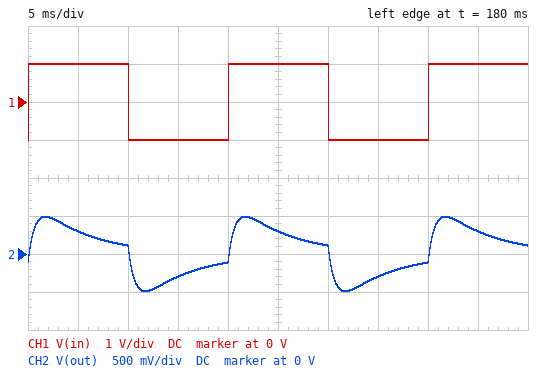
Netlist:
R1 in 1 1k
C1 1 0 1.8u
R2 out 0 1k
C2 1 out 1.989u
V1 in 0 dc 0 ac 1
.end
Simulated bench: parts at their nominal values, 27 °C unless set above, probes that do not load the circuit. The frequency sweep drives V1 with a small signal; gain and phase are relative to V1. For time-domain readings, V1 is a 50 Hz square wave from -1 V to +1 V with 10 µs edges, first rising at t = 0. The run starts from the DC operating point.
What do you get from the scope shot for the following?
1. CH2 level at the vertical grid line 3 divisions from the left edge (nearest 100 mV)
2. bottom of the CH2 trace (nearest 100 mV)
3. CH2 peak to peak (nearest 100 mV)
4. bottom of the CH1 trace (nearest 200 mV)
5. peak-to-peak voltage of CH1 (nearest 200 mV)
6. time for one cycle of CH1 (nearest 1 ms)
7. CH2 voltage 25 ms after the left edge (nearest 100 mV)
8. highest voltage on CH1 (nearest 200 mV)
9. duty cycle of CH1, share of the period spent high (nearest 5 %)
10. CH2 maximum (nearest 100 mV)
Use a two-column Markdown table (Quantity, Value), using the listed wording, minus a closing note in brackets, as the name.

| Quantity | Value |
|---|---|
| CH2 level at the vertical grid line 3 divisions from the left edge | -300 mV |
| bottom of the CH2 trace | -500 mV |
| CH2 peak to peak | 1.0 V |
| bottom of the CH1 trace | -1.0 V |
| peak-to-peak voltage of CH1 | 2.0 V |
| time for one cycle of CH1 | 20 ms |
| CH2 voltage 25 ms after the left edge | 300 mV |
| highest voltage on CH1 | 1.0 V |
| duty cycle of CH1, share of the period spent high | 50 % |
| CH2 maximum | 500 mV |
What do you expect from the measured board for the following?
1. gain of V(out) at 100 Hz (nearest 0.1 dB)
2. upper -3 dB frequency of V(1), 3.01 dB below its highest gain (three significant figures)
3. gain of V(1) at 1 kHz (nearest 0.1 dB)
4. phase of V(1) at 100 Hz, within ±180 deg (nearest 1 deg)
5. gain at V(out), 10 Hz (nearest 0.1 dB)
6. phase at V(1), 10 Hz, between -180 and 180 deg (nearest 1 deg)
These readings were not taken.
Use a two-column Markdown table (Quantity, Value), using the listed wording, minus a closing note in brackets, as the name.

| Quantity | Value |
|---|---|
| gain of V(out) at 100 Hz | -9.3 dB |
| upper -3 dB frequency of V(1), 3.01 dB below its highest gain | 36.5 Hz |
| gain of V(1) at 1 kHz | -21.3 dB |
| phase of V(1) at 100 Hz, within ±180 deg | -45 deg |
| gain at V(out), 10 Hz | -18.5 dB |
| phase at V(1), 10 Hz, between -180 and 180 deg | -13 deg |
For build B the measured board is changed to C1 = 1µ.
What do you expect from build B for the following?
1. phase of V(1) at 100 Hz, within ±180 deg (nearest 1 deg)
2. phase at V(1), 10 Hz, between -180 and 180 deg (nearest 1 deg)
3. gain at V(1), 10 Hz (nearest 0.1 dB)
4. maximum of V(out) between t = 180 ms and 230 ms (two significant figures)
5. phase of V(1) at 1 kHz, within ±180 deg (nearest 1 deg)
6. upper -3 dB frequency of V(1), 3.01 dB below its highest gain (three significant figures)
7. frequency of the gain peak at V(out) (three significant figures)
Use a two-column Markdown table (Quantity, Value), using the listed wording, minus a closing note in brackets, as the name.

| Quantity | Value |
|---|---|
| phase of V(1) at 100 Hz, within ±180 deg | -35 deg |
| phase at V(1), 10 Hz, between -180 and 180 deg | -10 deg |
| gain at V(1), 10 Hz | -0.3 dB |
| maximum of V(out) between t = 180 ms and 230 ms | 610 mV |
| phase of V(1) at 1 kHz, within ±180 deg | -73 deg |
| upper -3 dB frequency of V(1), 3.01 dB below its highest gain | 43.8 Hz |
| frequency of the gain peak at V(out) | 113 Hz |
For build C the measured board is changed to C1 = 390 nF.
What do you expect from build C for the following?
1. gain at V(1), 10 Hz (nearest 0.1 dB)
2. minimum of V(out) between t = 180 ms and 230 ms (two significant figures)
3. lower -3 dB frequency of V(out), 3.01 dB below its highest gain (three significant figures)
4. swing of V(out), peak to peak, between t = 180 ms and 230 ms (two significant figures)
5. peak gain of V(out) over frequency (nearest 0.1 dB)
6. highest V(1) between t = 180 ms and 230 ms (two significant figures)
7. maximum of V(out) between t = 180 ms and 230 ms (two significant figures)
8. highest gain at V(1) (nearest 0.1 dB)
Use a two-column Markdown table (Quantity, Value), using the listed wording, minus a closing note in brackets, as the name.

| Quantity | Value |
|---|---|
| gain at V(1), 10 Hz | -0.2 dB |
| minimum of V(out) between t = 180 ms and 230 ms | -750 mV |
| lower -3 dB frequency of V(out), 3.01 dB below its highest gain | 35.1 Hz |
| swing of V(out), peak to peak, between t = 180 ms and 230 ms | 1.5 V |
| peak gain of V(out) over frequency | -6.8 dB |
| highest V(1) between t = 180 ms and 230 ms | 910 mV |
| maximum of V(out) between t = 180 ms and 230 ms | 750 mV |
| highest gain at V(1) | 0 dB |
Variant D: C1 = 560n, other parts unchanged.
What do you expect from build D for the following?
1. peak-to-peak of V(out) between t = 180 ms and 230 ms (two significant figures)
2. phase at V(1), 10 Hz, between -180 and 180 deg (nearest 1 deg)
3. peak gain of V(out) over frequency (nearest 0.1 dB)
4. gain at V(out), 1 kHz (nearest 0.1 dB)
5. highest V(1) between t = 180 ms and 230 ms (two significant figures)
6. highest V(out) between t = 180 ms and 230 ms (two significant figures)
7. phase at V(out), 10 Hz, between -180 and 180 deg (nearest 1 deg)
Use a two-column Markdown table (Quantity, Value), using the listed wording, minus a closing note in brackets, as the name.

| Quantity | Value |
|---|---|
| peak-to-peak of V(out) between t = 180 ms and 230 ms | 1.4 V |
| phase at V(1), 10 Hz, between -180 and 180 deg | -9 deg |
| peak gain of V(out) over frequency | -7.2 dB |
| gain at V(out), 1 kHz | -12.3 dB |
| highest V(1) between t = 180 ms and 230 ms | 900 mV |
| highest V(out) between t = 180 ms and 230 ms | 700 mV |
| phase at V(out), 10 Hz, between -180 and 180 deg | 74 deg |
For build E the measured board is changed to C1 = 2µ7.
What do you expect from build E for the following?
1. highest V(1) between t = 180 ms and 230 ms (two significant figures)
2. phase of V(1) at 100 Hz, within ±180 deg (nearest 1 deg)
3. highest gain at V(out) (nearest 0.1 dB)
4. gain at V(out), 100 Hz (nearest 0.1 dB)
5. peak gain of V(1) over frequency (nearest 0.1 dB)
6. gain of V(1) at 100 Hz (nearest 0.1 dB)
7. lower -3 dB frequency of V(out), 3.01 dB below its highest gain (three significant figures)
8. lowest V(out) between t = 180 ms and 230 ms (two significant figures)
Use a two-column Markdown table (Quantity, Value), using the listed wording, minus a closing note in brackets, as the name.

| Quantity | Value |
|---|---|
| highest V(1) between t = 180 ms and 230 ms | 770 mV |
| phase of V(1) at 100 Hz, within ±180 deg | -54 deg |
| highest gain at V(out) | -10.5 dB |
| gain at V(out), 100 Hz | -10.8 dB |
| peak gain of V(1) over frequency | 0 dB |
| gain of V(1) at 100 Hz | -8.7 dB |
| lower -3 dB frequency of V(out), 3.01 dB below its highest gain | 21.5 Hz |
| lowest V(out) between t = 180 ms and 230 ms | -400 mV |
